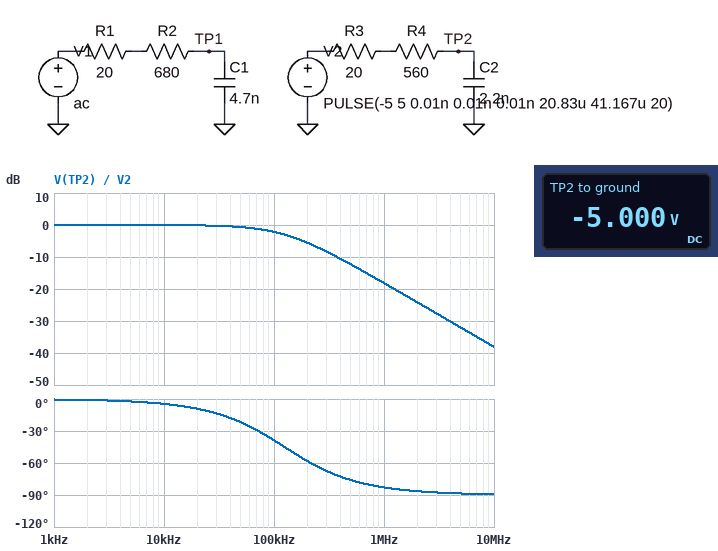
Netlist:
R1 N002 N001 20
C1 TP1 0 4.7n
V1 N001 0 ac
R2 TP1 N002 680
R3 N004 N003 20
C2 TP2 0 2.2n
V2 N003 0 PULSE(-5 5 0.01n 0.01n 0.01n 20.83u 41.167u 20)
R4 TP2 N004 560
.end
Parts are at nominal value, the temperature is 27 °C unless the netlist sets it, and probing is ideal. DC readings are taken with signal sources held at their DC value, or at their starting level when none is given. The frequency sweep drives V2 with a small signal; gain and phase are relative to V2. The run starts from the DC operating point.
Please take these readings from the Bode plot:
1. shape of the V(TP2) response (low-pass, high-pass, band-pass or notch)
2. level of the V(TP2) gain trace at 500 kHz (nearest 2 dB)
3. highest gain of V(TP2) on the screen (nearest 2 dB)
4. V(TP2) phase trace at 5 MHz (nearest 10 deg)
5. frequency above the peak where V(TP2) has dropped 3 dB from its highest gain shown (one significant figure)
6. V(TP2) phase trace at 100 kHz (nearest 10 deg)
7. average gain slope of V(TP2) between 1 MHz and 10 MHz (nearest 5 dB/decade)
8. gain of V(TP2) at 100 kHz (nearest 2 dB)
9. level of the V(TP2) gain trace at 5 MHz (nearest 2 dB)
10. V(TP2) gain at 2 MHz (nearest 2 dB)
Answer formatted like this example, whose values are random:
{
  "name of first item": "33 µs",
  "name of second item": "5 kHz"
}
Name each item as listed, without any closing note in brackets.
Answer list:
{
  "shape of the V(TP2) response": "low-pass",
  "level of the V(TP2) gain trace at 500 kHz": "-12 dB",
  "highest gain of V(TP2) on the screen": "0 dB",
  "V(TP2) phase trace at 5 MHz": "-90 deg",
  "frequency above the peak where V(TP2) has dropped 3 dB from its highest gain shown": "100 kHz",
  "V(TP2) phase trace at 100 kHz": "-40 deg",
  "average gain slope of V(TP2) between 1 MHz and 10 MHz": "-20 dB/decade",
  "gain of V(TP2) at 100 kHz": "-2 dB",
  "level of the V(TP2) gain trace at 5 MHz": "-32 dB",
  "V(TP2) gain at 2 MHz": "-24 dB"
}
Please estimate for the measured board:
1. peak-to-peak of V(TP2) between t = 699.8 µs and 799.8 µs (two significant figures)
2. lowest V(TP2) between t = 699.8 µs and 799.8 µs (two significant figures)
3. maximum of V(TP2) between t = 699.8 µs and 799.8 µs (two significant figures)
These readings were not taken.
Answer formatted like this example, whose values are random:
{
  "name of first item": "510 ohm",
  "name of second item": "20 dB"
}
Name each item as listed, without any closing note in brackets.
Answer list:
{
  "peak-to-peak of V(TP2) between t = 699.8 µs and 799.8 µs": "10 V",
  "lowest V(TP2) between t = 699.8 µs and 799.8 µs": "-5.0 V",
  "maximum of V(TP2) between t = 699.8 µs and 799.8 µs": "5.0 V"
}
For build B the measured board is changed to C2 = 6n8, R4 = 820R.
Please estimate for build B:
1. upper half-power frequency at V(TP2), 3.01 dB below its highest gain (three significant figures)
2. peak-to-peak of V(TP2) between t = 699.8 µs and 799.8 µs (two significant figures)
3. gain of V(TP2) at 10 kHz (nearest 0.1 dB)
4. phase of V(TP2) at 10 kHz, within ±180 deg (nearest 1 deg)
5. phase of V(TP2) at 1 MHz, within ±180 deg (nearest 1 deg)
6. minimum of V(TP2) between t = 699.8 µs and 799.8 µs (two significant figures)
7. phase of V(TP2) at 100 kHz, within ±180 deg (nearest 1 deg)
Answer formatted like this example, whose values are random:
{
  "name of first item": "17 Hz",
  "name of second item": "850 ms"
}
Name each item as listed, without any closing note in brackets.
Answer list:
{
  "upper half-power frequency at V(TP2), 3.01 dB below its highest gain": "27.9 kHz",
  "peak-to-peak of V(TP2) between t = 699.8 µs and 799.8 µs": "9.5 V",
  "gain of V(TP2) at 10 kHz": "-0.5 dB",
  "phase of V(TP2) at 10 kHz, within ±180 deg": "-20 deg",
  "phase of V(TP2) at 1 MHz, within ±180 deg": "-88 deg",
  "minimum of V(TP2) between t = 699.8 µs and 799.8 µs": "-4.7 V",
  "phase of V(TP2) at 100 kHz, within ±180 deg": "-74 deg"
}
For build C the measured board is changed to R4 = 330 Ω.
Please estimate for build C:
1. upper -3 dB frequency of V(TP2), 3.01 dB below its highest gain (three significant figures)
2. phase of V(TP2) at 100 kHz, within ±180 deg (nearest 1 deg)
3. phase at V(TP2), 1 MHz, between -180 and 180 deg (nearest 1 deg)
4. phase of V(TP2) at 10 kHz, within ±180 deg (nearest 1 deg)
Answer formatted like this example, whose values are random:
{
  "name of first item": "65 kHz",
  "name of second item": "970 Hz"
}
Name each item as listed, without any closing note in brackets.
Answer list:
{
  "upper -3 dB frequency of V(TP2), 3.01 dB below its highest gain": "207 kHz",
  "phase of V(TP2) at 100 kHz, within ±180 deg": "-26 deg",
  "phase at V(TP2), 1 MHz, between -180 and 180 deg": "-78 deg",
  "phase of V(TP2) at 10 kHz, within ±180 deg": "-3 deg"
}
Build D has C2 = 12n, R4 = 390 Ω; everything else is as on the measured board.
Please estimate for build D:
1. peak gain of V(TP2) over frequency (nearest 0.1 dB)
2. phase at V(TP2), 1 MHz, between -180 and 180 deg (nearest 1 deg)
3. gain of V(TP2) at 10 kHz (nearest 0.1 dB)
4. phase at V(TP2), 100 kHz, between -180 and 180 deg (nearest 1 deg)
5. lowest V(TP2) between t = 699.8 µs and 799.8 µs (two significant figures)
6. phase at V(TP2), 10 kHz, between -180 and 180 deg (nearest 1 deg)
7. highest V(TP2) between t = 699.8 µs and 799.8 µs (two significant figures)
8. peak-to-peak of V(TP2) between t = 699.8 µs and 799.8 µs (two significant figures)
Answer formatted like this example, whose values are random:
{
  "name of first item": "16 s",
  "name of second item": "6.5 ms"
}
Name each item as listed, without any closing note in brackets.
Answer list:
{
  "peak gain of V(TP2) over frequency": "0 dB",
  "phase at V(TP2), 1 MHz, between -180 and 180 deg": "-88 deg",
  "gain of V(TP2) at 10 kHz": "-0.4 dB",
  "phase at V(TP2), 100 kHz, between -180 and 180 deg": "-72 deg",
  "lowest V(TP2) between t = 699.8 µs and 799.8 µs": "-4.8 V",
  "phase at V(TP2), 10 kHz, between -180 and 180 deg": "-17 deg",
  "highest V(TP2) between t = 699.8 µs and 799.8 µs": "4.9 V",
  "peak-to-peak of V(TP2) between t = 699.8 µs and 799.8 µs": "9.7 V"
}
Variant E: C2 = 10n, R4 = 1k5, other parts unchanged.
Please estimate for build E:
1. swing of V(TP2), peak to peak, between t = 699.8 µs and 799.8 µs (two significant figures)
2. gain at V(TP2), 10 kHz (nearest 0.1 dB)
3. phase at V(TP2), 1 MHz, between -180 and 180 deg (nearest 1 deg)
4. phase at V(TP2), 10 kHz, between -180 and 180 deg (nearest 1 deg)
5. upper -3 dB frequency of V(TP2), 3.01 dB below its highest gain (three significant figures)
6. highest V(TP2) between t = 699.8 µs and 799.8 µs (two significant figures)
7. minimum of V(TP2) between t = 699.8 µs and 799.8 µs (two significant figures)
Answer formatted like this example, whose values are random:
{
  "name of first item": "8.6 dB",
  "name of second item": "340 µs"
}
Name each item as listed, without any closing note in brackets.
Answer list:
{
  "swing of V(TP2), peak to peak, between t = 699.8 µs and 799.8 µs": "5.9 V",
  "gain at V(TP2), 10 kHz": "-2.8 dB",
  "phase at V(TP2), 1 MHz, between -180 and 180 deg": "-89 deg",
  "phase at V(TP2), 10 kHz, between -180 and 180 deg": "-44 deg",
  "upper -3 dB frequency of V(TP2), 3.01 dB below its highest gain": "10.5 kHz",
  "highest V(TP2) between t = 699.8 µs and 799.8 µs": "3.0 V",
  "minimum of V(TP2) between t = 699.8 µs and 799.8 µs": "-2.9 V"
}
